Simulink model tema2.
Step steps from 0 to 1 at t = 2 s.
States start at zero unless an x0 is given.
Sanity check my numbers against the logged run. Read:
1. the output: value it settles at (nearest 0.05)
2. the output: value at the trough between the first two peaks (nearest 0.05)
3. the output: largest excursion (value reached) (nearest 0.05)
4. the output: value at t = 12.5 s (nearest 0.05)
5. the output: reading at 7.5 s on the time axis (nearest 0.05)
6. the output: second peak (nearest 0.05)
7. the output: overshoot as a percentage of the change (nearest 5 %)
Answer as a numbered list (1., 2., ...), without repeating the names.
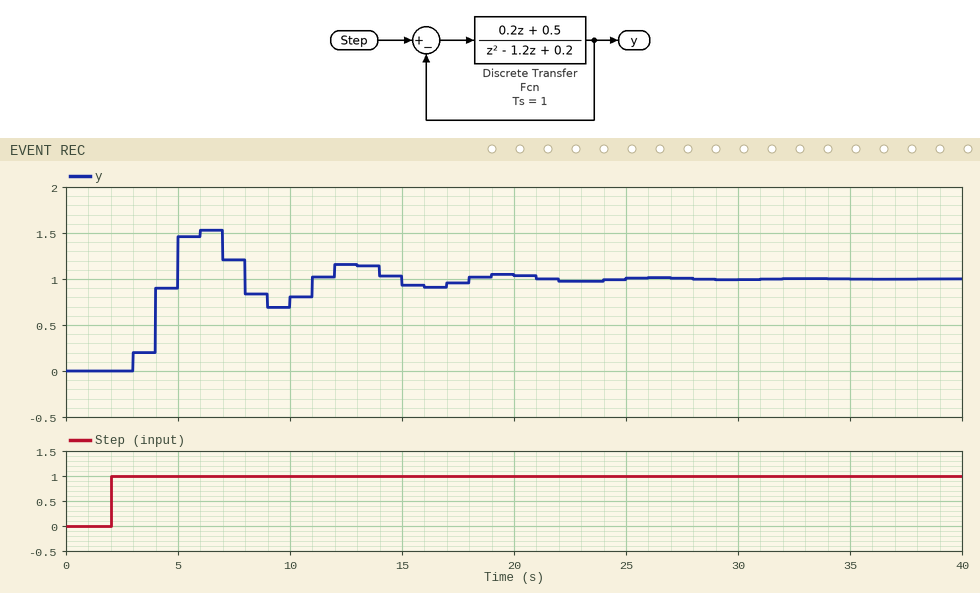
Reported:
1. 1.00
2. 0.70
3. 1.55
4. 1.15
5. 1.20
6. 1.15
7. 55 %
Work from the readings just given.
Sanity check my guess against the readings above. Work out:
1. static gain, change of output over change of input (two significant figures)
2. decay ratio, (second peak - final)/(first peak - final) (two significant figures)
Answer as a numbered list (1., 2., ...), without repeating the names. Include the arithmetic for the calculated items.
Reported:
1. (1 - 0) / (1 - 0) = 1.0
2. (1.15 - 1) / (1.55 - 1) = 0.27
